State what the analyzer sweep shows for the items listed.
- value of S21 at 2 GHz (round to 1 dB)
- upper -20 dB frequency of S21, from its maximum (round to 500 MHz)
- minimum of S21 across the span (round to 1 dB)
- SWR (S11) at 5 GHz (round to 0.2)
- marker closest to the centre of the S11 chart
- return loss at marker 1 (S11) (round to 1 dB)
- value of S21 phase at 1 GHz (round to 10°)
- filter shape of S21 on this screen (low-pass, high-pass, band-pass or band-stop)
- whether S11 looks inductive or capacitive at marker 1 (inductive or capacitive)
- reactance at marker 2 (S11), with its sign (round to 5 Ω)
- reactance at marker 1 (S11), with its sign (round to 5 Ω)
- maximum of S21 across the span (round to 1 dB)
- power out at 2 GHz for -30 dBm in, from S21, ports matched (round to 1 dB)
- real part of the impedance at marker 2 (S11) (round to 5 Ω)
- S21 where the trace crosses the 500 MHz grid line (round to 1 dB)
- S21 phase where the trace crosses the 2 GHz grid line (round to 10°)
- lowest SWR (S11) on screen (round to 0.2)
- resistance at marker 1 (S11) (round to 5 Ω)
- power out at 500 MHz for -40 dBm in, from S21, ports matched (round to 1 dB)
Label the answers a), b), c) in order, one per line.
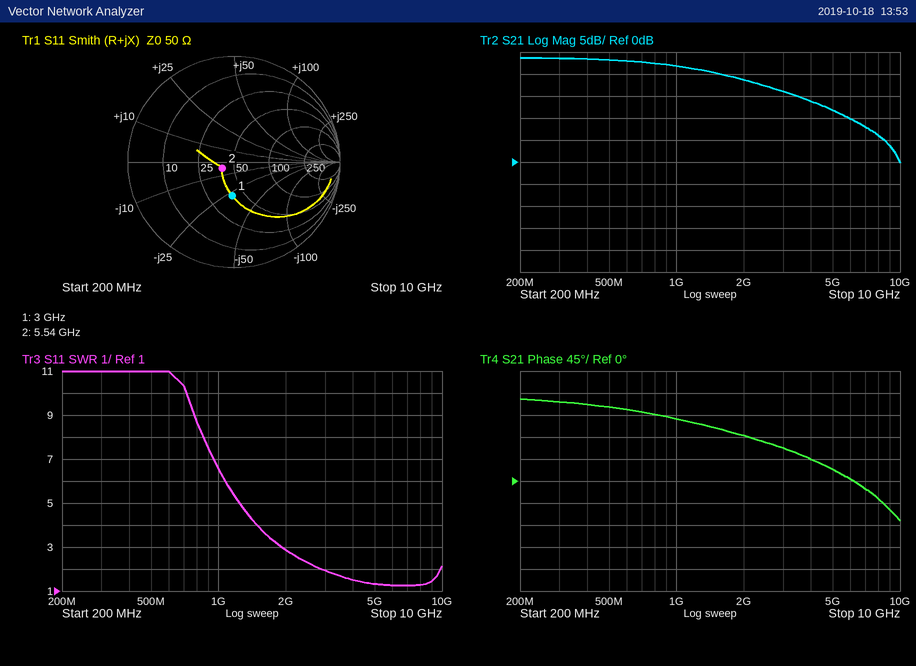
a) 19 dB
b) 9.0 GHz
c) 0 dB
d) 1.4
e) marker 2
f) 10 dB
g) 130°
h) low-pass
i) capacitive
j) -5 Ω
k) -30 Ω
l) 24 dB
m) -11 dBm
n) 40 Ω
o) 23 dB
p) 90°
q) 1.2
r) 40 Ω
s) -17 dBm
